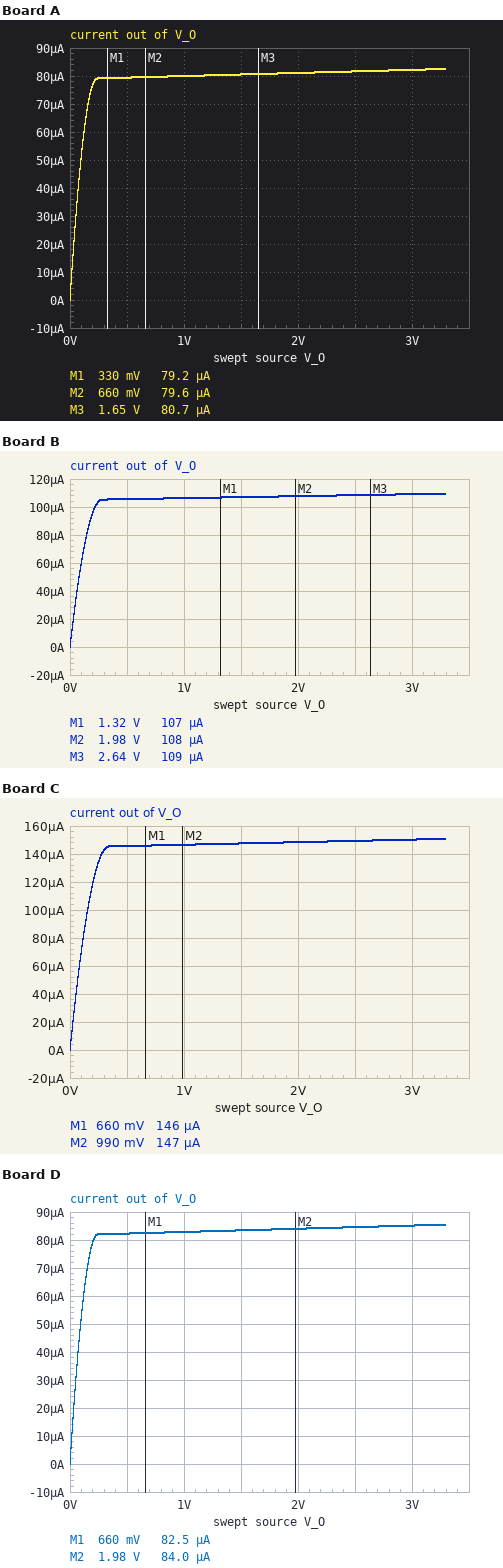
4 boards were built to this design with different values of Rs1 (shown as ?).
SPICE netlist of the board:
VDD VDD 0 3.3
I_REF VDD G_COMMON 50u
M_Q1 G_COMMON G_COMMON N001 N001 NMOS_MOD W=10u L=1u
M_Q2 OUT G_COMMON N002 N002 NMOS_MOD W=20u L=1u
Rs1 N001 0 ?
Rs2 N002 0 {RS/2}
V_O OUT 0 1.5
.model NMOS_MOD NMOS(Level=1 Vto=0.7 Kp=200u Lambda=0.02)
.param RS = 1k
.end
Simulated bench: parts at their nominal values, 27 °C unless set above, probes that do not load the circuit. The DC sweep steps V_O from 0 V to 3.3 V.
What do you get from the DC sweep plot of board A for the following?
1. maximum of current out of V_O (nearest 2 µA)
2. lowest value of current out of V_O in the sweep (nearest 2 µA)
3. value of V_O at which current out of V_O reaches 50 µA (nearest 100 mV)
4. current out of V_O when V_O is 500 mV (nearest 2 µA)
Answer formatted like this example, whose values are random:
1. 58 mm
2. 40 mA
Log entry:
1. 82 µA
2. 0 A
3. 100 mV
4. 80 µA
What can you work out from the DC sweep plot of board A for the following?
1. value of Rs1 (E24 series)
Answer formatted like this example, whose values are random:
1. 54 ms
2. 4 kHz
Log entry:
1. 330 Ω
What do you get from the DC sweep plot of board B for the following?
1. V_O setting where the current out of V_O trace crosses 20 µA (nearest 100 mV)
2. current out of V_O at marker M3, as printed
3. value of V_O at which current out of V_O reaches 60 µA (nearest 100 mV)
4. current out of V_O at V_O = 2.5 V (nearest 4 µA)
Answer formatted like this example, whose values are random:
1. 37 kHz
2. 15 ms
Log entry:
1. 0 V
2. 109 µA
3. 100 mV
4. 108 µA
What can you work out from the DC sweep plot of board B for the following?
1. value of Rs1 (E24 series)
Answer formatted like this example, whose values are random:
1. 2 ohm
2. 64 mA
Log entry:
1. 1.2 kΩ
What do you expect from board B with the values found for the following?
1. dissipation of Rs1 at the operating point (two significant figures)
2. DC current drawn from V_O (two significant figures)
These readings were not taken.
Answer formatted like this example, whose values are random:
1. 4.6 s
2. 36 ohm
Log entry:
1. 3.0 µW
2. 110 µA
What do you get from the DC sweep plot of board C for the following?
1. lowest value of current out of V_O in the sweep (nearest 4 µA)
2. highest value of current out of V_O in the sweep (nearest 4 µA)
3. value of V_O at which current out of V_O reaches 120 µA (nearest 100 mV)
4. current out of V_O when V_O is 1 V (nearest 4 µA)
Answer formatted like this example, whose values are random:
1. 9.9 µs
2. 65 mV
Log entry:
1. 0 A
2. 152 µA
3. 200 mV
4. 148 µA
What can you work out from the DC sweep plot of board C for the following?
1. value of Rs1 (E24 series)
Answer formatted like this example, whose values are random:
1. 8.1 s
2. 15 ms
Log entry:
1. 2.4 kΩ
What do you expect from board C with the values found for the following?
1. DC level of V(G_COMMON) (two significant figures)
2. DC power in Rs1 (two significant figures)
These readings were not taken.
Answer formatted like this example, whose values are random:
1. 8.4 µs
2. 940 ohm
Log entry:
1. 1.0 V
2. 6.0 µW
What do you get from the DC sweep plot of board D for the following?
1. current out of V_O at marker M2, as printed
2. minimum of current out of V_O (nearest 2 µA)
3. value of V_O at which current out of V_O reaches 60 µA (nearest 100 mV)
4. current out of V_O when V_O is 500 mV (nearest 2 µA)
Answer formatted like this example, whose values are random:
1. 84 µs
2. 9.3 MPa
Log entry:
1. 84.0 µA
2. 0 A
3. 100 mV
4. 82 µA
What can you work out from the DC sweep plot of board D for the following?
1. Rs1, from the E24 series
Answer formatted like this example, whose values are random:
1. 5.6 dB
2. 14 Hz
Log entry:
1. 430 Ω
